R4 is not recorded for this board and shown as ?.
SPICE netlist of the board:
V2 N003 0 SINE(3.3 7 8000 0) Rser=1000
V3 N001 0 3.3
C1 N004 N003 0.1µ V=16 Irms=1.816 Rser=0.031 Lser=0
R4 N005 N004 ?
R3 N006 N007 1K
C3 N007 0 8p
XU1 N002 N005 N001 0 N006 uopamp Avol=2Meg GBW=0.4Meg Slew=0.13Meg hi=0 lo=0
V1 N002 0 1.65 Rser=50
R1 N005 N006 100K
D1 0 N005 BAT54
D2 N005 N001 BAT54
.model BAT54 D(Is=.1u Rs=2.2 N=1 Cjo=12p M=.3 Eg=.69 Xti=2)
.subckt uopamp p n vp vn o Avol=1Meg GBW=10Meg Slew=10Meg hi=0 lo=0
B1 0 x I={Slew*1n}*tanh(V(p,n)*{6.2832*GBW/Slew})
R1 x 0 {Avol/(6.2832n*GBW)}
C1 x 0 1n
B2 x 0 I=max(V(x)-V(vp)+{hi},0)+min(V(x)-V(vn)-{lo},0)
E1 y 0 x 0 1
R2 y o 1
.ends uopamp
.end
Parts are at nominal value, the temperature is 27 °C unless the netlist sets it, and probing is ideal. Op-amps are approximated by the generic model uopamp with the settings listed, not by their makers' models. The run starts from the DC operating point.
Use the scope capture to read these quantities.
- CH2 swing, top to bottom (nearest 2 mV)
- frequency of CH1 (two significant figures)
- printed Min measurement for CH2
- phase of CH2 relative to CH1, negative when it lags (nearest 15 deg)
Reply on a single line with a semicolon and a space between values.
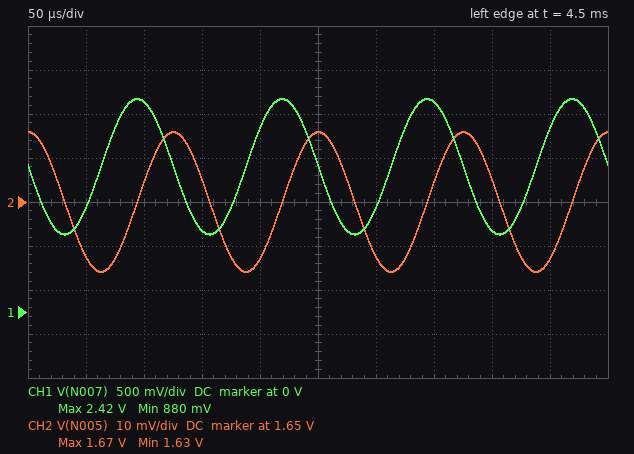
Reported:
32 mV; 8.0 kHz; 1.63 V; -90 deg
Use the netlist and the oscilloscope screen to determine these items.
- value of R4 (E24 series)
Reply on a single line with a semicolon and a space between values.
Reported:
910 kΩ
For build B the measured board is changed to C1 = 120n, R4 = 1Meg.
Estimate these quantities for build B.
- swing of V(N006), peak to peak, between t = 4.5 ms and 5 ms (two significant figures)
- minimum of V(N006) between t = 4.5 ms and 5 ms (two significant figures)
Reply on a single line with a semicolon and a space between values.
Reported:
1.4 V; 950 mV
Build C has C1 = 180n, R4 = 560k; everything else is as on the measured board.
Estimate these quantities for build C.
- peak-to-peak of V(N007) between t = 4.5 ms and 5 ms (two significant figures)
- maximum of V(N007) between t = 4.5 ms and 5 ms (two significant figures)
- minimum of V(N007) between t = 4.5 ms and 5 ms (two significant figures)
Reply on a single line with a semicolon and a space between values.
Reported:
2.5 V; 2.9 V; 400 mV
